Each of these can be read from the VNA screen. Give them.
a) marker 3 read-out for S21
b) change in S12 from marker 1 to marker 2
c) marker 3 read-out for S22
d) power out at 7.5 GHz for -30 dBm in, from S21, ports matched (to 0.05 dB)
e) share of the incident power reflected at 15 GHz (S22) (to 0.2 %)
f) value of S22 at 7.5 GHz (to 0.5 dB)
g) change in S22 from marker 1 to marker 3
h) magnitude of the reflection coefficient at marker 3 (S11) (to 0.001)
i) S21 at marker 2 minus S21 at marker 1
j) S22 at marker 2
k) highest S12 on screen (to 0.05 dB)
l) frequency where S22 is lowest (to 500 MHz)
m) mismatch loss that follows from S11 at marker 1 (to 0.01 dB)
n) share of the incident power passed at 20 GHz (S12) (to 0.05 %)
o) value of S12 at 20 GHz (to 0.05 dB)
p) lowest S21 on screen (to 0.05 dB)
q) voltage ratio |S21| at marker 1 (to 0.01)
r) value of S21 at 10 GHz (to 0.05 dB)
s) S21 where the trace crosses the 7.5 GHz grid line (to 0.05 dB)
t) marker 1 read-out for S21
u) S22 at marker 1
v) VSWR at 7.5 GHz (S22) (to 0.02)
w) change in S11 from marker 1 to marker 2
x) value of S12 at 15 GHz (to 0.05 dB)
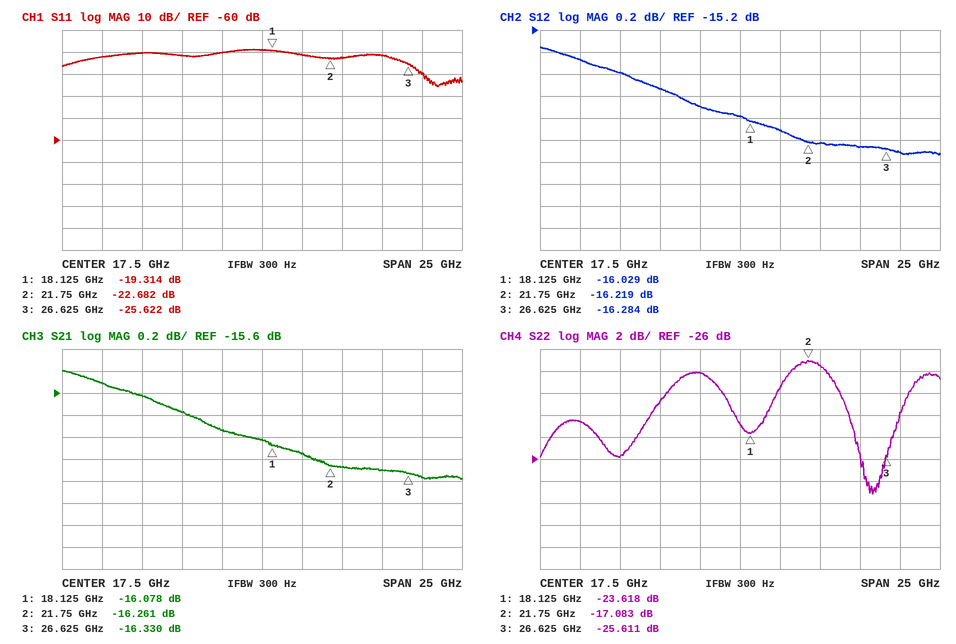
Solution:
-16.330 dB
-0.190 dB
-25.611 dB
-45.50 dBm
1.6 %
-22.5 dB
-1.993 dB
0.052
-0.183 dB
-17.083 dB
-15.35 dB
26.0 GHz
0.05 dB
2.45 %
-16.10 dB
-16.40 dB
0.16
-15.60 dB
-15.50 dB
-16.078 dB
-23.618 dB
1.16
-3.368 dB
-15.90 dB
